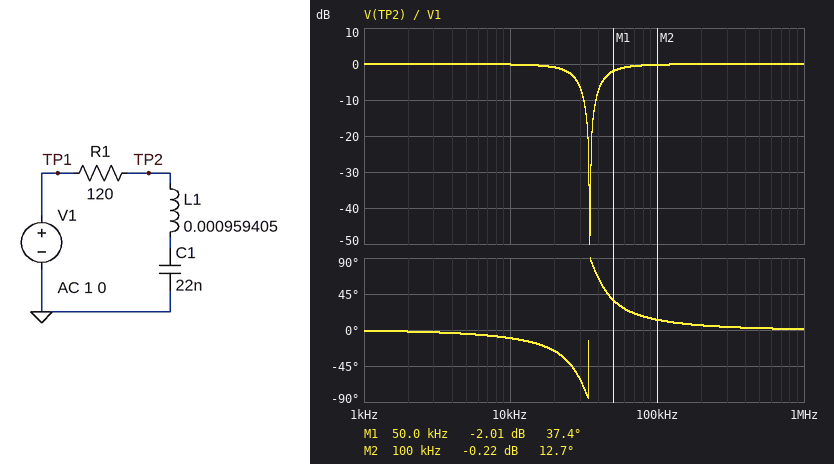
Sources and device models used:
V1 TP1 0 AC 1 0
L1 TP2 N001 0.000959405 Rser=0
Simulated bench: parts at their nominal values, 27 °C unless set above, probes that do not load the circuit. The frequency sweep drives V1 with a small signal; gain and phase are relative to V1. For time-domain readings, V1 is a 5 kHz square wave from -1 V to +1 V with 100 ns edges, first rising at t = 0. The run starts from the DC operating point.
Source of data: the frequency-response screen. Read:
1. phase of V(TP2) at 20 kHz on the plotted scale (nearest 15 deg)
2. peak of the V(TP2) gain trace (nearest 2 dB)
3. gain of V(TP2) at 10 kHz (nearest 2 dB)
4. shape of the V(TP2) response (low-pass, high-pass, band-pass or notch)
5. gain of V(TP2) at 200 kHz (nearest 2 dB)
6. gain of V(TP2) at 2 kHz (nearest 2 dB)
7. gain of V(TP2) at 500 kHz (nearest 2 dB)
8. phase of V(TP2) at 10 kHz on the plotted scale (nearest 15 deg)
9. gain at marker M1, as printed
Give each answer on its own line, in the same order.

-30 deg
0 dB
0 dB
notch
0 dB
0 dB
0 dB
-15 deg
-2.01 dB
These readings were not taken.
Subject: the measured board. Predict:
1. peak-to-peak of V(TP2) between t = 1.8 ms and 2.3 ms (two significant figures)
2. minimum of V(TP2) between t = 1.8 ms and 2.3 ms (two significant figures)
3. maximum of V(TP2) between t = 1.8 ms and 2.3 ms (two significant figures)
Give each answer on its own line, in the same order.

2.6 V
-1.3 V
1.3 V
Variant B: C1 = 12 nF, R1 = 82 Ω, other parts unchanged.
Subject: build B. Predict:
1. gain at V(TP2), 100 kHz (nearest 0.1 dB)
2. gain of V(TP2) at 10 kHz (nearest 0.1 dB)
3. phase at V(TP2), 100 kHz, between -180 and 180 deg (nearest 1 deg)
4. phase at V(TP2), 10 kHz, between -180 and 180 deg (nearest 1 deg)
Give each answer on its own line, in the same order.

-0.1 dB
0 dB
10 deg
-4 deg
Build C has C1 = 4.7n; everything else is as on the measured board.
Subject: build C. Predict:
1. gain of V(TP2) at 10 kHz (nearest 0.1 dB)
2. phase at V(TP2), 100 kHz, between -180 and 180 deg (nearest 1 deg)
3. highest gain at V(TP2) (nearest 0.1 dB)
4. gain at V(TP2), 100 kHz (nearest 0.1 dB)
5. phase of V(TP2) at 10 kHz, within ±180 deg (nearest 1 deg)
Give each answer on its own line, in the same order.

0 dB
24 deg
0 dB
-0.8 dB
-2 deg
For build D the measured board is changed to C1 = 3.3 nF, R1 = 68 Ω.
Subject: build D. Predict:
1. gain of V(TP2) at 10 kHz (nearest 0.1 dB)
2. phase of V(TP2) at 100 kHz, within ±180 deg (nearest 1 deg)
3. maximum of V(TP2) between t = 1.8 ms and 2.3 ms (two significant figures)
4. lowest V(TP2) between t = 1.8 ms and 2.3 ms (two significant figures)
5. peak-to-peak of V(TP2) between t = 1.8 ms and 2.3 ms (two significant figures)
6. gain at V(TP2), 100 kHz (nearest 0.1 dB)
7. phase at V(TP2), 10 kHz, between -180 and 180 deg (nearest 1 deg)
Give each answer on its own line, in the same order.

0 dB
29 deg
1.2 V
-1.2 V
2.4 V
-1.2 dB
-1 deg
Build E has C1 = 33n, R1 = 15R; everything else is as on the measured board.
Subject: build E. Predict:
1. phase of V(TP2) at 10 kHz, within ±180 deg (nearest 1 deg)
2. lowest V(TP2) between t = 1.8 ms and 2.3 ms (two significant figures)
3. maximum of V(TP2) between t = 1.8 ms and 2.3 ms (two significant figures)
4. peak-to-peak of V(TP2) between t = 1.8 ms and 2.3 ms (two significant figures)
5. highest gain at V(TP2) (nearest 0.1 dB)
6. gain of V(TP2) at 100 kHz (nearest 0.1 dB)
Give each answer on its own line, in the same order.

-2 deg
-1.1 V
1.1 V
2.2 V
0 dB
0 dB
